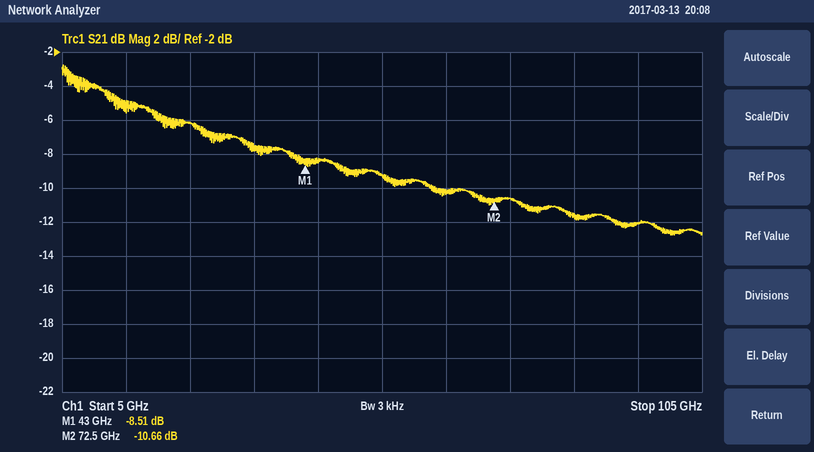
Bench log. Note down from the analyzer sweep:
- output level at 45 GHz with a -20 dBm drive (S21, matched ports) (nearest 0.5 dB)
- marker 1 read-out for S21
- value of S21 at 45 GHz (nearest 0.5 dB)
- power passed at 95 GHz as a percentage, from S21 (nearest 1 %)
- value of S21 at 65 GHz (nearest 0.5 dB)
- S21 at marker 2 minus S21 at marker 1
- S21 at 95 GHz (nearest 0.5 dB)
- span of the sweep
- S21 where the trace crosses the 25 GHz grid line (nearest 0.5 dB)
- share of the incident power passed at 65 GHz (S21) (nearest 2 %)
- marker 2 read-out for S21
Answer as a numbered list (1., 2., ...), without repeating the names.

1. -28.5 dBm
2. -8.51 dB
3. -8.5 dB
4. 6 %
5. -10.0 dB
6. -2.15 dB
7. -12.0 dB
8. 100 GHz
9. -6.0 dB
10. 10 %
11. -10.66 dB
